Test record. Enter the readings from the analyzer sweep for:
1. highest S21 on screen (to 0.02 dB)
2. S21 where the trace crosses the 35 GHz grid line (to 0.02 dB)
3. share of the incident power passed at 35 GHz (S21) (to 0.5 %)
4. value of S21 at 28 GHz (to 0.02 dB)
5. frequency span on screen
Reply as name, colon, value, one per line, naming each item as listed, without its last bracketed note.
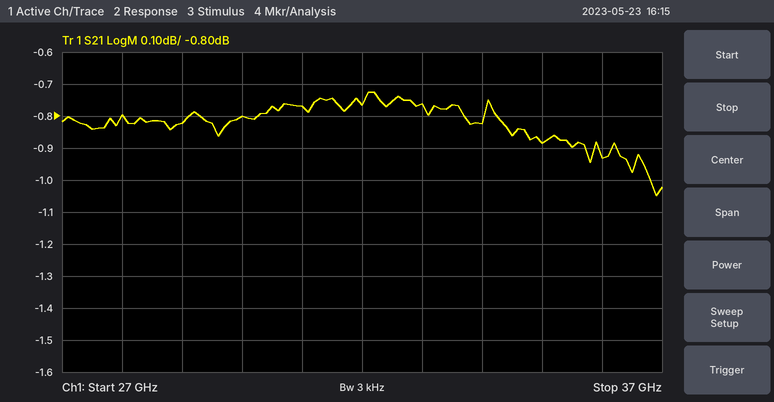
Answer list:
highest S21 on screen: -0.72 dB
S21 where the trace crosses the 35 GHz grid line: -0.88 dB
share of the incident power passed at 35 GHz (S21): 81.5 %
value of S21 at 28 GHz: -0.80 dB
frequency span on screen: 10 GHz
